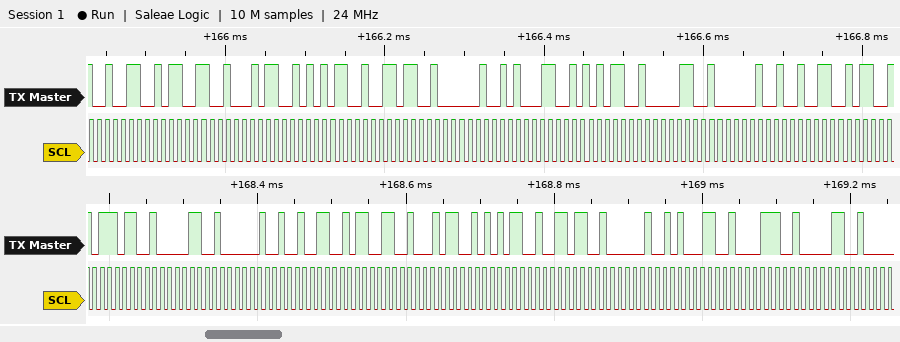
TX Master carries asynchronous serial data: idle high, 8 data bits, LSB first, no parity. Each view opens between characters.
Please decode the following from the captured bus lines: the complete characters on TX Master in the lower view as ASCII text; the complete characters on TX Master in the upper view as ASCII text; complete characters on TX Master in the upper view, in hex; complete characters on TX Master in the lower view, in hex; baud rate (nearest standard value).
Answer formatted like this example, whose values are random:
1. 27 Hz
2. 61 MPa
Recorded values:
1. "70 23456 180"
2. "23456 150 2"
3. 32, 33, 34, 35, 36, 20, 31, 35, 30, 20, 32
4. 37, 30, 20, 32, 33, 34, 35, 36, 20, 31, 38, 30
5. 115200 baud
